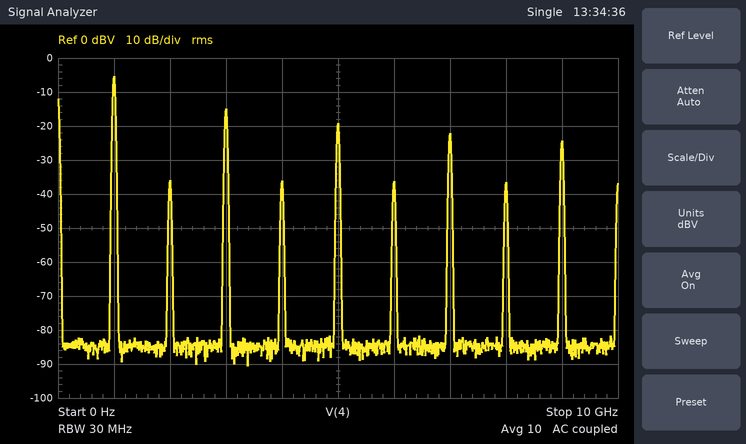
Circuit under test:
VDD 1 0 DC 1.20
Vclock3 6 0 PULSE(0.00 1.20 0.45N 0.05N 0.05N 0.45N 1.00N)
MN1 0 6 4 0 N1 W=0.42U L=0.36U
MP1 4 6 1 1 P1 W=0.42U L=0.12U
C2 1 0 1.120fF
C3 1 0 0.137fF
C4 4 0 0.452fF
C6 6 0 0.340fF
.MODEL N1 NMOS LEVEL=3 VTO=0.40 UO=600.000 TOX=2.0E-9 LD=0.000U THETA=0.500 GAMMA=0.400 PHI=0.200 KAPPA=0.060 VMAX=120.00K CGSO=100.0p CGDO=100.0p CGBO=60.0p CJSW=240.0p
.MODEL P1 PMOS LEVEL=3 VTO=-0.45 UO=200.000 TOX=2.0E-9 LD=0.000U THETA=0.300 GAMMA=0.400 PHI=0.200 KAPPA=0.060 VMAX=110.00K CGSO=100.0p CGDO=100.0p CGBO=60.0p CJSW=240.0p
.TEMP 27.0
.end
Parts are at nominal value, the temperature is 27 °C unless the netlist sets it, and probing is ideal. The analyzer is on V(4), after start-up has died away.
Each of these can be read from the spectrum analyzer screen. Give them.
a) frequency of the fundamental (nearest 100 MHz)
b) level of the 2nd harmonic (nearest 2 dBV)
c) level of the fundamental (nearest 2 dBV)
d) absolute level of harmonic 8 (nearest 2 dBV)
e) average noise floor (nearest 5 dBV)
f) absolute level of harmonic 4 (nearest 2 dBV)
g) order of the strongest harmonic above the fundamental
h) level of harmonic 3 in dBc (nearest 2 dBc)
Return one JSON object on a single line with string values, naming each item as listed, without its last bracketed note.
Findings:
{"frequency of the fundamental": "1.0 GHz", "level of the 2nd harmonic": "-36 dBV", "level of the fundamental": "-6 dBV", "absolute level of harmonic 8": "-36 dBV", "average noise floor": "-85 dBV", "absolute level of harmonic 4": "-36 dBV", "order of the strongest harmonic above the fundamental": "3", "level of harmonic 3 in dBc": "-10 dBc"}
